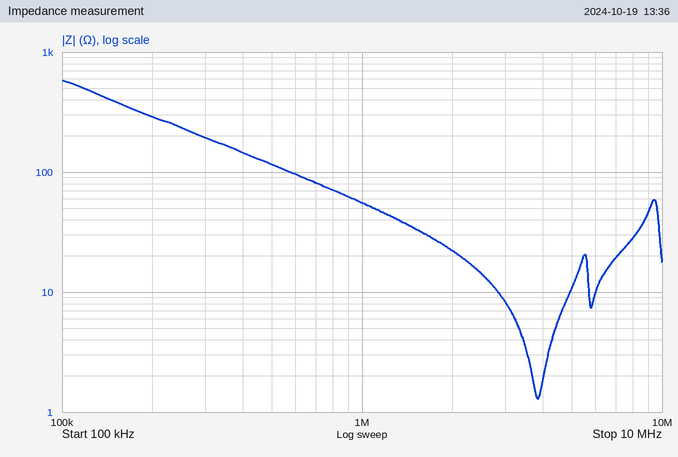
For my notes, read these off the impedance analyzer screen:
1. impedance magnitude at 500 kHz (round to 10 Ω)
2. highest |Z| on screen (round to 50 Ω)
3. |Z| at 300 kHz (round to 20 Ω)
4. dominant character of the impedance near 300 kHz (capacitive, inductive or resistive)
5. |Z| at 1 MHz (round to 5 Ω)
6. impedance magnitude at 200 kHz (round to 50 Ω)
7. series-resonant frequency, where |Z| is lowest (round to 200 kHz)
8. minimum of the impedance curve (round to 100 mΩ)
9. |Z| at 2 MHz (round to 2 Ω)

120 Ω
600 Ω
200 Ω
capacitive
55 Ω
300 Ω
3.8 MHz
1.3 Ω
22 Ω
